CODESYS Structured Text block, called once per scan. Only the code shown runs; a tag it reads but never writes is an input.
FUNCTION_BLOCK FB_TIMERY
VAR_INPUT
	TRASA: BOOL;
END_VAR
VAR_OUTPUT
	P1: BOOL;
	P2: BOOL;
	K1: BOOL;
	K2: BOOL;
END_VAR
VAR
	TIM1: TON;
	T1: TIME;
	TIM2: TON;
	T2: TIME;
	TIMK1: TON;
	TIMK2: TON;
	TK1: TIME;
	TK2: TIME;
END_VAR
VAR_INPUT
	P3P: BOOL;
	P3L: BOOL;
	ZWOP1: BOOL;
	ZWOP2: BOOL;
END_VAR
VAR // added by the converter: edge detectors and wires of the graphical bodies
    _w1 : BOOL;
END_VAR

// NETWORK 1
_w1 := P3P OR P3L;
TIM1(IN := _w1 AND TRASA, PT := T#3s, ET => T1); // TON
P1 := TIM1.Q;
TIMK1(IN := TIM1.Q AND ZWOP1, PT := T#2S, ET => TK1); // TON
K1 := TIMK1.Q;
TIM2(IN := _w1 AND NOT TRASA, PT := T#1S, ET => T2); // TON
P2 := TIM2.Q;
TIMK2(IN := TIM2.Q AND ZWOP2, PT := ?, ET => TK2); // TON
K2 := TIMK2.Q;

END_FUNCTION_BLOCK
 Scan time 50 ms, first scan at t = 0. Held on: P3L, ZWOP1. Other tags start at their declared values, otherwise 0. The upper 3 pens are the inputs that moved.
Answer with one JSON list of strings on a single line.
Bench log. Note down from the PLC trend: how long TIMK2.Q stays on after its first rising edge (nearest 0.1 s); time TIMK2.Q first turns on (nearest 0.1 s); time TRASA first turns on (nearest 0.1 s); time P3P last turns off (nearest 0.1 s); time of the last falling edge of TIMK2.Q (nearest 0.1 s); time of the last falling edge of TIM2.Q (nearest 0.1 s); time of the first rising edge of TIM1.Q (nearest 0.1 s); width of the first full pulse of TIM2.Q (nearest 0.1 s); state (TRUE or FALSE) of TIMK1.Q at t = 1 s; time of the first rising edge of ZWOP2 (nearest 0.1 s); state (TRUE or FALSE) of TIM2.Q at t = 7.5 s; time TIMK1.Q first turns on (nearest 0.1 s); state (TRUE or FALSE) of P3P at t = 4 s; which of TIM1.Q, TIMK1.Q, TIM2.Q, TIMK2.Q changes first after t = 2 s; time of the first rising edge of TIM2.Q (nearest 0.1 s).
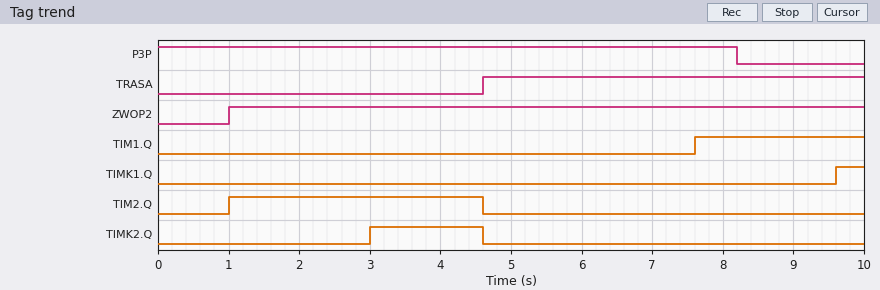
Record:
["1.6 s", "3.0 s", "4.6 s", "8.2 s", "4.6 s", "4.6 s", "7.6 s", "3.6 s", "FALSE", "1.0 s", "FALSE", "9.6 s", "TRUE", "TIMK2.Q", "1.0 s"]
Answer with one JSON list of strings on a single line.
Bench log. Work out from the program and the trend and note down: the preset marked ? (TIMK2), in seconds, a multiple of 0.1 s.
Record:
["2.0 s"]
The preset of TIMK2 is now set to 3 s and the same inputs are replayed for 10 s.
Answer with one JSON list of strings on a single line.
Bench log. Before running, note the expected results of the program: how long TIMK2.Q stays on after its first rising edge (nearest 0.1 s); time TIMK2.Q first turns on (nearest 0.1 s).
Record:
["0.6 s", "4.0 s"]
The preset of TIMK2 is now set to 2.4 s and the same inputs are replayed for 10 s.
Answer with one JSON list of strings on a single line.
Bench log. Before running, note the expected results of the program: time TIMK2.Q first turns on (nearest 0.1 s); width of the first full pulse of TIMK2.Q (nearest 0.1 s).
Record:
["3.4 s", "1.2 s"]
